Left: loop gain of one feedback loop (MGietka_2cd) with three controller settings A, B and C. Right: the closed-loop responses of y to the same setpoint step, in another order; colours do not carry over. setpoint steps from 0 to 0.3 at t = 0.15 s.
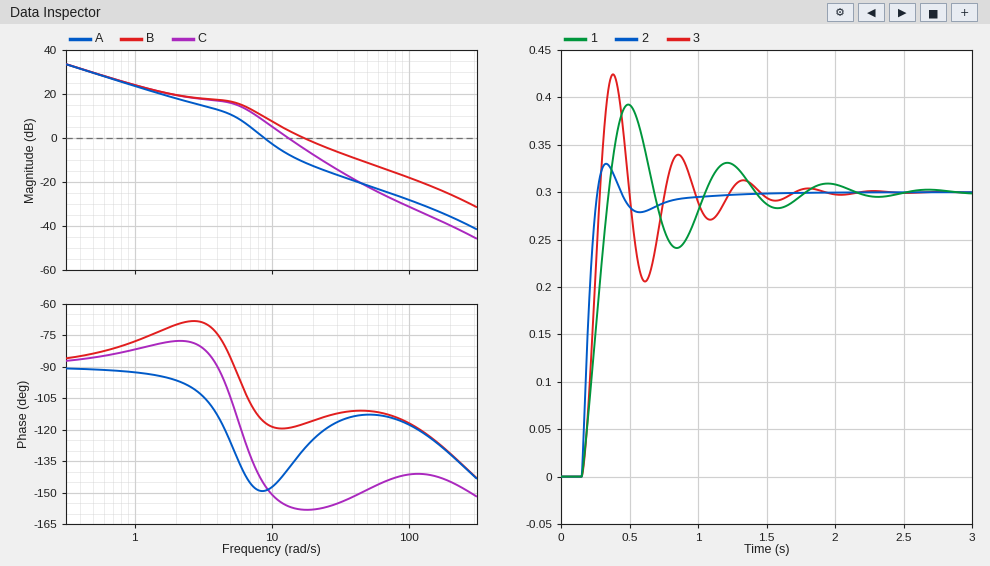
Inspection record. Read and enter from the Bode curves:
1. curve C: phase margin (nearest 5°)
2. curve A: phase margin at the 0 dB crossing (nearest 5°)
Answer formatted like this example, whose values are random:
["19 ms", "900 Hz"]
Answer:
["25°", "30°"]
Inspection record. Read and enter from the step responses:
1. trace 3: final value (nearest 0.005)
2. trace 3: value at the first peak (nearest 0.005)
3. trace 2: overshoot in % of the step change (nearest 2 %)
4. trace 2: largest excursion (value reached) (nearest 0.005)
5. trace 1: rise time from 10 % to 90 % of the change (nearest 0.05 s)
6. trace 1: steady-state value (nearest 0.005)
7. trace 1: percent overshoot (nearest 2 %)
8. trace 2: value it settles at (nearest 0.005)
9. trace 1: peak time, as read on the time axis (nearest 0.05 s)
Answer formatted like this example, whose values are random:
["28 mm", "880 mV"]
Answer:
["0.300", "0.425", "10 %", "0.330", "0.15 s", "0.300", "30 %", "0.300", "0.50 s"]
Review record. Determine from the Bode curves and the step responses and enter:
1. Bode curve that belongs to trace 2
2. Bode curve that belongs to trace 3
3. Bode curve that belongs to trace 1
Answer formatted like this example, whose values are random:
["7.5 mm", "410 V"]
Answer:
["B", "C", "A"]
